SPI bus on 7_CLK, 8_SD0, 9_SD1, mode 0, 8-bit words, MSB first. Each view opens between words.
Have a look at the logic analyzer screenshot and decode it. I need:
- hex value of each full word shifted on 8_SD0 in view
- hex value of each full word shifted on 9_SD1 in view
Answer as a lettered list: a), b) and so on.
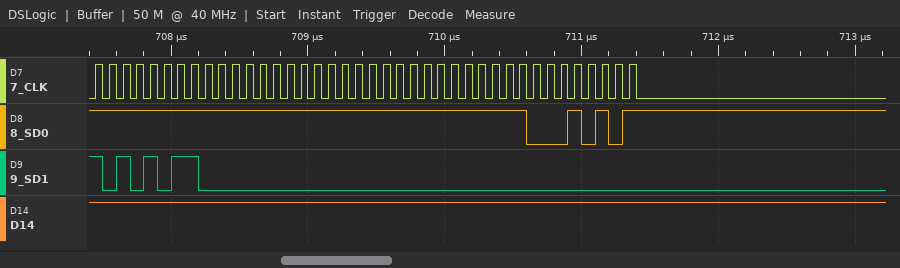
a) FF, FF, FF, FF, 15
b) AB, 00, 00, 00, 00
